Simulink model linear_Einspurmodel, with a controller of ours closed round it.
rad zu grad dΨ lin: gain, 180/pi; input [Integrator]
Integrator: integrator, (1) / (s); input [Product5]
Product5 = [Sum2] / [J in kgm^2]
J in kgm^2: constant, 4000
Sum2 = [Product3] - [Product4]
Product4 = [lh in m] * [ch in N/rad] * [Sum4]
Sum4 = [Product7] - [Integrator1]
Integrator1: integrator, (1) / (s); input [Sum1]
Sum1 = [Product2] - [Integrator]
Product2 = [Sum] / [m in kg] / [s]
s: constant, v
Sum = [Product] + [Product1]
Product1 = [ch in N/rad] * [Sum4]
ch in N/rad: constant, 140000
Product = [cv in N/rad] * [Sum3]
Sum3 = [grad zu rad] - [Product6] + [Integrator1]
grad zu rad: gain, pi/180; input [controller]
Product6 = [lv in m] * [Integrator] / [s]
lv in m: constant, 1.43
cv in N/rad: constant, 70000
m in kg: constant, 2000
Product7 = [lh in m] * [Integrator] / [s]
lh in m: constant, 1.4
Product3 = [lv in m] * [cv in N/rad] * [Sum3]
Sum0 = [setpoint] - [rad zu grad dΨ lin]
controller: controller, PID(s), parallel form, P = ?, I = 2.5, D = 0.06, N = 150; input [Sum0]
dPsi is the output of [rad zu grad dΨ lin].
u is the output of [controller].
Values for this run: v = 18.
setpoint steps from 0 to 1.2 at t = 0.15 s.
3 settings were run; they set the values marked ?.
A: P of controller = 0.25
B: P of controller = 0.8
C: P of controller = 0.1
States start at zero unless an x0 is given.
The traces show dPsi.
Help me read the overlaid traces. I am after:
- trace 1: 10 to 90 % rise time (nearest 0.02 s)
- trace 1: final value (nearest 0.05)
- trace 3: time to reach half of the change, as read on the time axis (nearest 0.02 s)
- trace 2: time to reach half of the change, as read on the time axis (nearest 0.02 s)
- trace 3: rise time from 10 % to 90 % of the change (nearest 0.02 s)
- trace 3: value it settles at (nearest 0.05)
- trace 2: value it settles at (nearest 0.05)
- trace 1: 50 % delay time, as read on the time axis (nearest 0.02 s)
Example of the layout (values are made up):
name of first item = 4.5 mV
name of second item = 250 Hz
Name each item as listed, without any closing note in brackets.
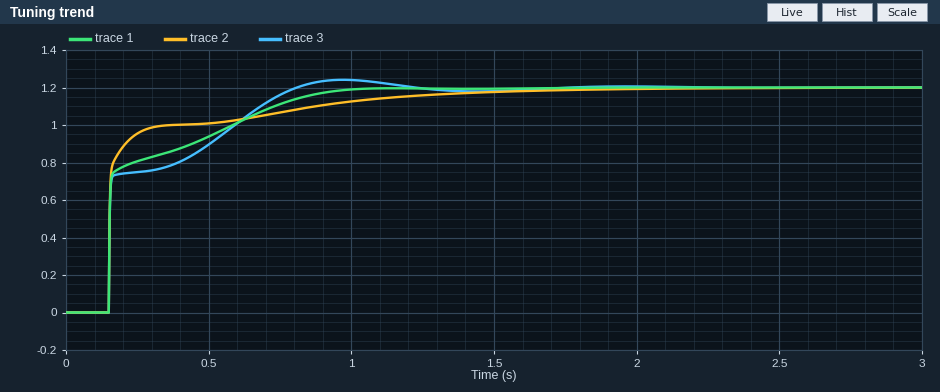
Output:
trace 1: 10 to 90 % rise time = 0.54 s
trace 1: final value = 1.20
trace 3: time to reach half of the change, as read on the time axis = 0.16 s
trace 2: time to reach half of the change, as read on the time axis = 0.16 s
trace 3: rise time from 10 % to 90 % of the change = 0.52 s
trace 3: value it settles at = 1.20
trace 2: value it settles at = 1.20
trace 1: 50 % delay time, as read on the time axis = 0.16 s
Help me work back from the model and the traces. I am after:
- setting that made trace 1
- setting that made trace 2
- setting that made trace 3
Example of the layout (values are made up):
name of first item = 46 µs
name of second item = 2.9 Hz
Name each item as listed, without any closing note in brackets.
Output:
setting that made trace 1 = A
setting that made trace 2 = B
setting that made trace 3 = C
